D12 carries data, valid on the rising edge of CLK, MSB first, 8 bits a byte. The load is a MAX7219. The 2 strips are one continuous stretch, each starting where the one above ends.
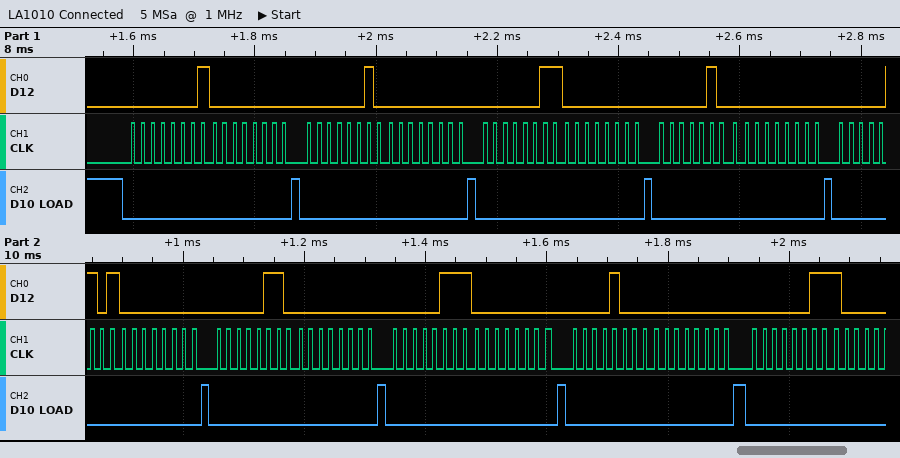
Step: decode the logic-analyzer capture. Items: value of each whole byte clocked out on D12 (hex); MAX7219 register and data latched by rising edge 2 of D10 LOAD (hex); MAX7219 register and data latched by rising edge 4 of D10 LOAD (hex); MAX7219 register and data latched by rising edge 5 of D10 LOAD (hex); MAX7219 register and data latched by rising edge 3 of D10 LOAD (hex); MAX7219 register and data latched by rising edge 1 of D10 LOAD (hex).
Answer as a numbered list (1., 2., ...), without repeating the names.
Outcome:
1. 01 00 02 00 03 00 04 00 05 00 06 00 07 00 08 00 03
2. register 0x2, data 0x00
3. register 0x4, data 0x00
4. register 0x5, data 0x00
5. register 0x3, data 0x00
6. register 0x1, data 0x00
